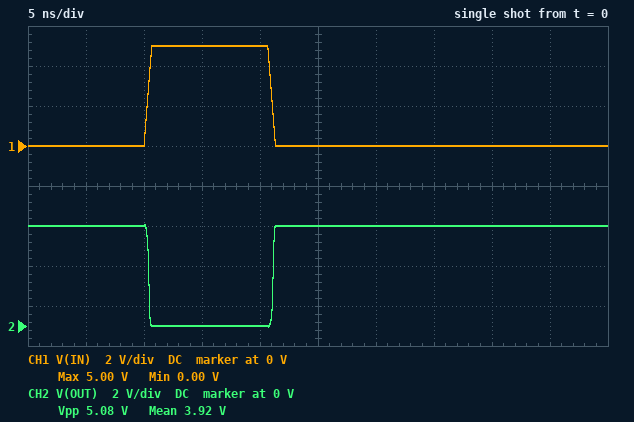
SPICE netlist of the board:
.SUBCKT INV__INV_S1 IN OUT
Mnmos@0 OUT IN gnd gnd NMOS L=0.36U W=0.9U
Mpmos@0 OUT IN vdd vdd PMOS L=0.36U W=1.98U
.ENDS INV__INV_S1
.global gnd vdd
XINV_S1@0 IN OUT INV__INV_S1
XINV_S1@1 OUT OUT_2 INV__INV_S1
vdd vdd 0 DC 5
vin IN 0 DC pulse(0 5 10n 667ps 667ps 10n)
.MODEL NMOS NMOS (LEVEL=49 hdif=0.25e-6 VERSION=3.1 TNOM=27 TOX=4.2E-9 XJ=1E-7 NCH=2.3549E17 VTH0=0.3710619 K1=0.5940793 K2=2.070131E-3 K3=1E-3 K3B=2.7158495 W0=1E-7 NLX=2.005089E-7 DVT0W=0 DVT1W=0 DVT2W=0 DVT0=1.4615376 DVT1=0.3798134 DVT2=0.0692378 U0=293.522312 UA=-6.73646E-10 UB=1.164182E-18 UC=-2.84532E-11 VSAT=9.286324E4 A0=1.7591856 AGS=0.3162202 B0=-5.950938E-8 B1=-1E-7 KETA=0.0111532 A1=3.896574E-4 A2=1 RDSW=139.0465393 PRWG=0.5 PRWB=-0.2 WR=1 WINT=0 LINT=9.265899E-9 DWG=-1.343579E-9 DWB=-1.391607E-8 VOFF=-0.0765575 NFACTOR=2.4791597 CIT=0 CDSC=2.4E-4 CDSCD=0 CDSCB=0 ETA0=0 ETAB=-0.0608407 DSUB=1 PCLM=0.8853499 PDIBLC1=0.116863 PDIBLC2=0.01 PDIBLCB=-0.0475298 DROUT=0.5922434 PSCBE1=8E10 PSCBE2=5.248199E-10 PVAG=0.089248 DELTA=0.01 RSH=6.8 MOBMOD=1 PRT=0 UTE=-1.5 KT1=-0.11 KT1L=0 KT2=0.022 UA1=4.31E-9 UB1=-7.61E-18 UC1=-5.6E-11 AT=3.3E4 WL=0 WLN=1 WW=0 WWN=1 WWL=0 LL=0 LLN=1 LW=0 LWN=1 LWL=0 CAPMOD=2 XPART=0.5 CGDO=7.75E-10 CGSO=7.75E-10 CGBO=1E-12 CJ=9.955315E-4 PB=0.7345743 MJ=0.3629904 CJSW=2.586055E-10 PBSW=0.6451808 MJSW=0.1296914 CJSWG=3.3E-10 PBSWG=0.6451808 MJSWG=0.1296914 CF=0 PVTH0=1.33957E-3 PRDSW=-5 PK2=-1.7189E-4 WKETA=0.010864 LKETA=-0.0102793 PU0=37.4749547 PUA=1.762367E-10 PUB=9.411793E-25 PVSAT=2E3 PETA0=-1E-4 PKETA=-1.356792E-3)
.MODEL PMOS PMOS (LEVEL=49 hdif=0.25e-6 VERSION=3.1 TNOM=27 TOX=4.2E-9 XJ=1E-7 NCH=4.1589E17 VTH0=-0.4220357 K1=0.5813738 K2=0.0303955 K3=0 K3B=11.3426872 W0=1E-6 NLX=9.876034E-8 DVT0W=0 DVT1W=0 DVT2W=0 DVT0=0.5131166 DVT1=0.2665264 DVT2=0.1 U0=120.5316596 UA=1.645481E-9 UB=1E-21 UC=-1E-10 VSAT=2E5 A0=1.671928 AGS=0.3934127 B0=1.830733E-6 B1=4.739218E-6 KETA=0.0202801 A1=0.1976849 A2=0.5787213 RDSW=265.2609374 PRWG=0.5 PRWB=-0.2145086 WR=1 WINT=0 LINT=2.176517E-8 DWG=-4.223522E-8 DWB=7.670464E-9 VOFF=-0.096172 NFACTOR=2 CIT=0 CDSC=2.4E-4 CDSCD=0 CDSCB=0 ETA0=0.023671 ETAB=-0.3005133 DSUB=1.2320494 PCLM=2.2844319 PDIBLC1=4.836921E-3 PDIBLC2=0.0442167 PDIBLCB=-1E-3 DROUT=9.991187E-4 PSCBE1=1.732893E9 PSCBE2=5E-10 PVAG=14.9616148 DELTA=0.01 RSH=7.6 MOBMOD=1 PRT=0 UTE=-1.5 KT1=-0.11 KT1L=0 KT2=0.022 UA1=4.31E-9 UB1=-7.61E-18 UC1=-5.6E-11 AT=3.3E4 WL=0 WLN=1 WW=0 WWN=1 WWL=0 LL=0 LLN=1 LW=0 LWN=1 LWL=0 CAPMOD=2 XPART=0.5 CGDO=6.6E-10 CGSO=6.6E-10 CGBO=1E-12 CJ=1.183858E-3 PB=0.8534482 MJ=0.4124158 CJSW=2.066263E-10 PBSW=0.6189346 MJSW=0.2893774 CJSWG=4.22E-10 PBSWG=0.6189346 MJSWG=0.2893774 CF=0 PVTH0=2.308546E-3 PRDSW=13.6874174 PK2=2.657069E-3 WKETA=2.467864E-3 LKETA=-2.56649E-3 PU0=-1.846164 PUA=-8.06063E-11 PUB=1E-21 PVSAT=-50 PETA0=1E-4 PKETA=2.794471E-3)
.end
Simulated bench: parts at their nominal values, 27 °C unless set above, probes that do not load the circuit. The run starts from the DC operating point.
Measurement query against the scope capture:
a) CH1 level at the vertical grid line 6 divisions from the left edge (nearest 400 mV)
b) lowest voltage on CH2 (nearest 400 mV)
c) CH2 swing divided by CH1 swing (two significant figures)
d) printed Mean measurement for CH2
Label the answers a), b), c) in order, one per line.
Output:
a) 0 V
b) 0 V
c) 1.0
d) 3.92 V
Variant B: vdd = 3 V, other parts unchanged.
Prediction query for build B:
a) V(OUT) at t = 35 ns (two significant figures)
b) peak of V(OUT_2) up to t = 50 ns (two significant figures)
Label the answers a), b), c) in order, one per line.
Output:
a) 3.0 V
b) 3.1 V
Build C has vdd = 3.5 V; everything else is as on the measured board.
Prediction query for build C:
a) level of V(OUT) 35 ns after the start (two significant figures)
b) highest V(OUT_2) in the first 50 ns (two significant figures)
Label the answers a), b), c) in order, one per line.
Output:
a) 3.5 V
b) 3.6 V
